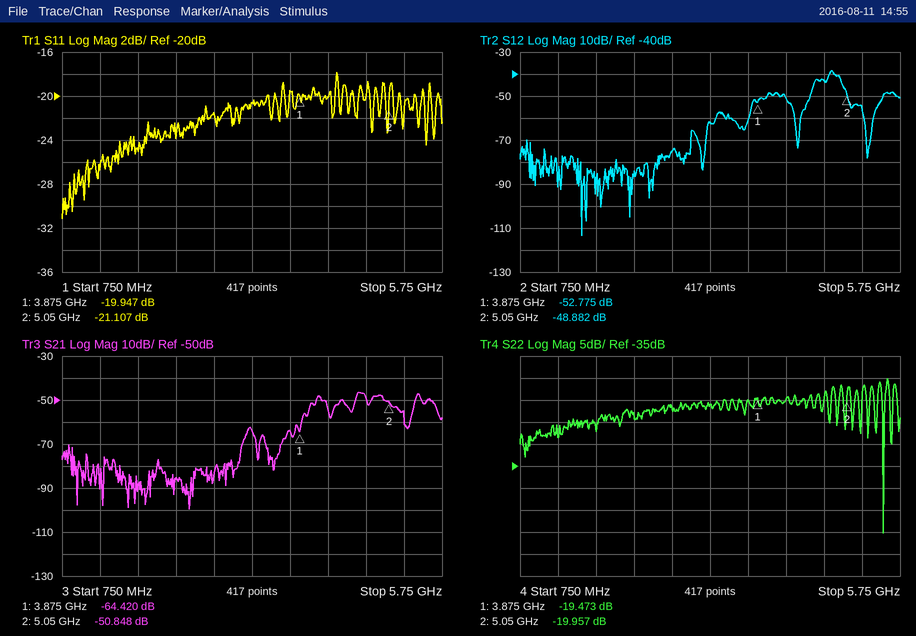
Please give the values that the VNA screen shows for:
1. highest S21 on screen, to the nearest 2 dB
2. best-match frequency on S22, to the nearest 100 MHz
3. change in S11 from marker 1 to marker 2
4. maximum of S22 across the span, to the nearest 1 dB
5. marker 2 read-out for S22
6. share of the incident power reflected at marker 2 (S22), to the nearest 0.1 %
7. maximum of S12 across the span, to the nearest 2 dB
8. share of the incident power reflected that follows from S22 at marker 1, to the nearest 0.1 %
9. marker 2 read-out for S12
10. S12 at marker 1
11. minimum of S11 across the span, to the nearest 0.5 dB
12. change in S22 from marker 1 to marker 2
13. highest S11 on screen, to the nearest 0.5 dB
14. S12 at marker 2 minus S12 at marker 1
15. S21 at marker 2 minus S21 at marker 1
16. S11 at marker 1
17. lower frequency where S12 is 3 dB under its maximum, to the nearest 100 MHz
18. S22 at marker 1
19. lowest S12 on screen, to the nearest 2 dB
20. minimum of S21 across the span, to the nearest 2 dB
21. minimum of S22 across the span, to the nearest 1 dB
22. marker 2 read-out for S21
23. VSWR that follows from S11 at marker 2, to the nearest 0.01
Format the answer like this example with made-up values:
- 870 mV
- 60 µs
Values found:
- -46 dB
- 5.5 GHz
- -1.160 dB
- -15 dB
- -19.957 dB
- 1.0 %
- -38 dB
- 1.1 %
- -48.882 dB
- -52.775 dB
- -31.0 dB
- -0.484 dB
- -18.0 dB
- 3.893 dB
- 13.572 dB
- -19.947 dB
- 4.8 GHz
- -19.473 dB
- -114 dB
- -100 dB
- -50 dB
- -50.848 dB
- 1.19
